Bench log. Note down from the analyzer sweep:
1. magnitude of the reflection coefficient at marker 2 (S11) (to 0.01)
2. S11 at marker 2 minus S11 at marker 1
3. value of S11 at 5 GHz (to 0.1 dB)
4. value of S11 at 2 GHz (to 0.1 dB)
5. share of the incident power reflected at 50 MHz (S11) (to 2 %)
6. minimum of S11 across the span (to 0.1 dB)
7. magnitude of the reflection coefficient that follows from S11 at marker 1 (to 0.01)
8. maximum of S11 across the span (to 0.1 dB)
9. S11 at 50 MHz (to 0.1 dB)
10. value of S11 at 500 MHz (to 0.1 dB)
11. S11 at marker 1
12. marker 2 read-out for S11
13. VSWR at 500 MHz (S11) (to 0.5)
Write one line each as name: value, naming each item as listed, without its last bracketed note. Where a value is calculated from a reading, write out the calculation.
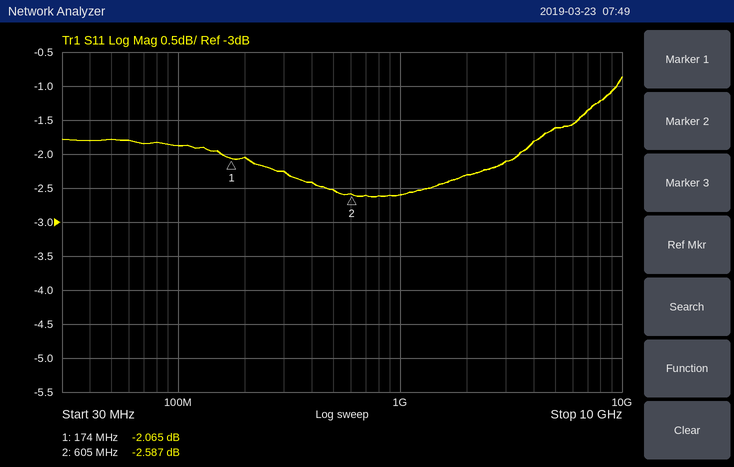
magnitude of the reflection coefficient at marker 2 (S11): 10^(-2.587/20) ≈ 0.74
S11 at marker 2 minus S11 at marker 1: -2.587 − (-2.065) = -0.522 dB
value of S11 at 5 GHz: -1.6 dB
value of S11 at 2 GHz: -2.3 dB
share of the incident power reflected at 50 MHz (S11): 10^(-1.8/10) ≈ 66 %
minimum of S11 across the span: -2.6 dB
magnitude of the reflection coefficient that follows from S11 at marker 1: 10^(-2.065/20) ≈ 0.79
maximum of S11 across the span: -0.9 dB
S11 at 50 MHz: -1.8 dB
value of S11 at 500 MHz: -2.5 dB
S11 at marker 1: -2.065 dB
marker 2 read-out for S11: -2.587 dB
VSWR at 500 MHz (S11): |Γ| = 10^(-2.5/20) = 0.7499; VSWR = (1 + 0.7499)/(1 − 0.7499) ≈ 7.0
